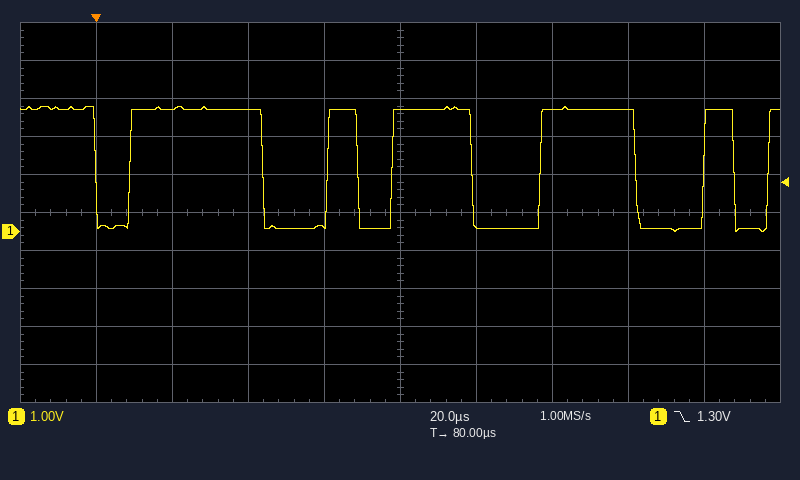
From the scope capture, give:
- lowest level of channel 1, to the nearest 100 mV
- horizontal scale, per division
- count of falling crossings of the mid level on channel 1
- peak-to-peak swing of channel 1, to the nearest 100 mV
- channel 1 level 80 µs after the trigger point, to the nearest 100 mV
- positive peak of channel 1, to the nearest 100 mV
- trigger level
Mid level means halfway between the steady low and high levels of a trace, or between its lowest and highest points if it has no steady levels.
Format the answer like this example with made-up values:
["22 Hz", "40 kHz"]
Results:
["0.0 V", "20 µs", "6", "3.3 V", "3.2 V", "3.3 V", "1.30 V"]
